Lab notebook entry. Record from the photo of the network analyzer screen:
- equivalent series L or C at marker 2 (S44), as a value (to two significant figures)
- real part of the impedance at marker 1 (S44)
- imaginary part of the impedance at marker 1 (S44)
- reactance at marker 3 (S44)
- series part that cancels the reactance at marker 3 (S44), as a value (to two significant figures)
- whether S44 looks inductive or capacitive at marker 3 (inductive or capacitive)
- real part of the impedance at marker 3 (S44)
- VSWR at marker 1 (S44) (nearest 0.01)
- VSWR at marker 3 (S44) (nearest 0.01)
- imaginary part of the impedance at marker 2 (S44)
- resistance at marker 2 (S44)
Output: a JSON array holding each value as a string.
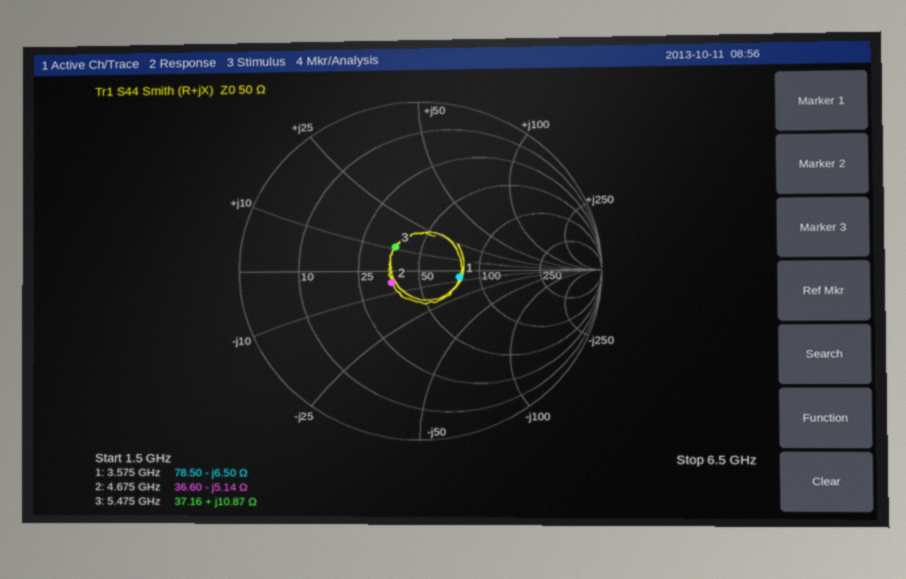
["6.6 pF", "78.50 Ω", "-6.50 Ω", "+10.87 Ω", "2.7 pF", "inductive", "37.16 Ω", "1.59", "1.47", "-5.14 Ω", "36.60 Ω"]
